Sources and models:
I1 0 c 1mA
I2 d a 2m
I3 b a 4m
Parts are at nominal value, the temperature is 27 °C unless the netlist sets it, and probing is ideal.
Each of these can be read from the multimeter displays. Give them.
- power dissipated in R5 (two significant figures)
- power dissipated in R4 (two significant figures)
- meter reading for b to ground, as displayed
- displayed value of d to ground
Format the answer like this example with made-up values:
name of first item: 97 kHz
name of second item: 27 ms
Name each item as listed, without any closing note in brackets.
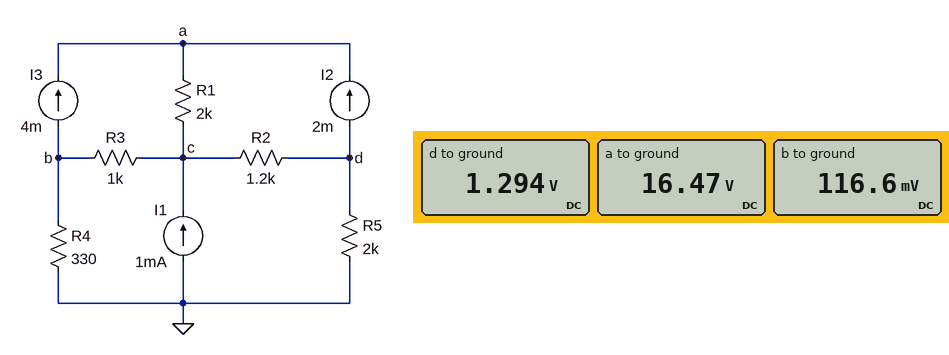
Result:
power dissipated in R5: 840 µW
power dissipated in R4: 41 µW
meter reading for b to ground, as displayed: 116.6 mV
displayed value of d to ground: 1.294 V
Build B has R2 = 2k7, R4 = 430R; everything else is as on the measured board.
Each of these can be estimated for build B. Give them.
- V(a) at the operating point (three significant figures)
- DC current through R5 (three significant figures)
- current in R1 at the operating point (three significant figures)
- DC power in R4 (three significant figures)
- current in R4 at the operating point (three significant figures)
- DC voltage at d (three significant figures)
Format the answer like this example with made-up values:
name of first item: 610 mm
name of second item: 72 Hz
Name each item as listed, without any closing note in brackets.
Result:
V(a) at the operating point: 17.4 V
DC current through R5: 4.89 µA
current in R1 at the operating point: 6.00 mA
DC power in R4: 426 µW
current in R4 at the operating point: 995 µA
DC voltage at d: 9.79 mV
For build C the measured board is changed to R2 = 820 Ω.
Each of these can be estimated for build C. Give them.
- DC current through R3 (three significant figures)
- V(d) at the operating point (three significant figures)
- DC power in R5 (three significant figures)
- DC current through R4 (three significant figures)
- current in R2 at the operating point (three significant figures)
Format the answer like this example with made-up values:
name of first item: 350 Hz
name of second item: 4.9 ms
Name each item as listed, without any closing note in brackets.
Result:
DC current through R3: 4.11 mA
V(d) at the operating point: 1.78 V
DC power in R5: 1.58 mW
DC current through R4: 111 µA
current in R2 at the operating point: 2.89 mA
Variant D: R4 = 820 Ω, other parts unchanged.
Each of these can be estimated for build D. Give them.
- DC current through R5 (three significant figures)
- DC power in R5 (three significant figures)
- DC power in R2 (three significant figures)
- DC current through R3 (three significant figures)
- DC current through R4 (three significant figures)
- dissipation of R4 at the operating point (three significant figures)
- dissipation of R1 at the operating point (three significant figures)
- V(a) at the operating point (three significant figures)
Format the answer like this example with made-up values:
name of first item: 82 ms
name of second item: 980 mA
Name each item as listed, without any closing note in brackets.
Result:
DC current through R5: 681 µA
DC power in R5: 928 µW
DC power in R2: 8.63 mW
DC current through R3: 4.32 mA
DC current through R4: 319 µA
dissipation of R4 at the operating point: 83.3 µW
dissipation of R1 at the operating point: 72.0 mW
V(a) at the operating point: 16.6 V
